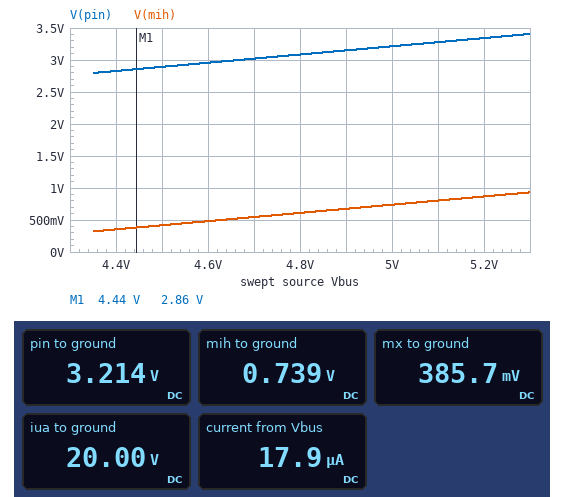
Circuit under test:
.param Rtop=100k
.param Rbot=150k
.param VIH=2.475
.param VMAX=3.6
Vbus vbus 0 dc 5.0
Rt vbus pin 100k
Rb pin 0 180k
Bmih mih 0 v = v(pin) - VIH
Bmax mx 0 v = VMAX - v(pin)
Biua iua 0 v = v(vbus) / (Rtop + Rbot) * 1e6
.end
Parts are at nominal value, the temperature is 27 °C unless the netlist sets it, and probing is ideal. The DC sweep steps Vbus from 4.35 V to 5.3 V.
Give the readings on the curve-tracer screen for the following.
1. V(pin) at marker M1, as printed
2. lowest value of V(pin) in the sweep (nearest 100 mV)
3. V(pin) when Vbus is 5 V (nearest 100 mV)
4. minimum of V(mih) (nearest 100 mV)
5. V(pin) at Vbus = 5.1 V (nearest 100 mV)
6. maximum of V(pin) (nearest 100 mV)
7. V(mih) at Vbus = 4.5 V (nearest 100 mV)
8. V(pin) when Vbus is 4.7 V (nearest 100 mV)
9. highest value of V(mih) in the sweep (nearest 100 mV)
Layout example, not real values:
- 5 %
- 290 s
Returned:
- 2.86 V
- 2.8 V
- 3.2 V
- 300 mV
- 3.3 V
- 3.4 V
- 400 mV
- 3.0 V
- 900 mV
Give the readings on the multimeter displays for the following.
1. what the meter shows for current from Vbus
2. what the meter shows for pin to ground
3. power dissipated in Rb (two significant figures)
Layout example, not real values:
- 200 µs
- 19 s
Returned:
- 17.9 µA
- 3.214 V
- 57 µW
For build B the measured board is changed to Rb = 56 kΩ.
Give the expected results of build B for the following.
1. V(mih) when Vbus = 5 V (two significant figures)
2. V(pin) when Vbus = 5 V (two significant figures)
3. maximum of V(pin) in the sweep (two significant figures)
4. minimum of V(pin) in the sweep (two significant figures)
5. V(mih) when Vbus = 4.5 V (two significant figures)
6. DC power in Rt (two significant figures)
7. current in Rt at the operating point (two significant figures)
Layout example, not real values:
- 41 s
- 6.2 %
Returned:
- -680 mV
- 1.8 V
- 1.9 V
- 1.6 V
- -860 mV
- 100 µW
- 32 µA
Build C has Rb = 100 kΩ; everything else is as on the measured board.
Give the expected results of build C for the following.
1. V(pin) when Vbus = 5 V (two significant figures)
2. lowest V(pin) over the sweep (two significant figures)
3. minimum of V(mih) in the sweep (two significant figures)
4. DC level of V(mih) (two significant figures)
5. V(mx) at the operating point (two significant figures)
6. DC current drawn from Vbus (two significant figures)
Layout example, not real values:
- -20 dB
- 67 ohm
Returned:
- 2.5 V
- 2.2 V
- -300 mV
- 25 mV
- 1.1 V
- 25 µA
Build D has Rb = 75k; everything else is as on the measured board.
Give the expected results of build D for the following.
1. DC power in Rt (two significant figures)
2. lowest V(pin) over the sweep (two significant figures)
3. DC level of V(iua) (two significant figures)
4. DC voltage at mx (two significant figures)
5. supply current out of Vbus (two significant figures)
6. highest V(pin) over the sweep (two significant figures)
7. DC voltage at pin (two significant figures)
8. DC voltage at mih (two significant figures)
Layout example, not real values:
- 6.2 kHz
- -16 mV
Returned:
- 82 µW
- 1.9 V
- 20 V
- 1.5 V
- 29 µA
- 2.3 V
- 2.1 V
- -330 mV
